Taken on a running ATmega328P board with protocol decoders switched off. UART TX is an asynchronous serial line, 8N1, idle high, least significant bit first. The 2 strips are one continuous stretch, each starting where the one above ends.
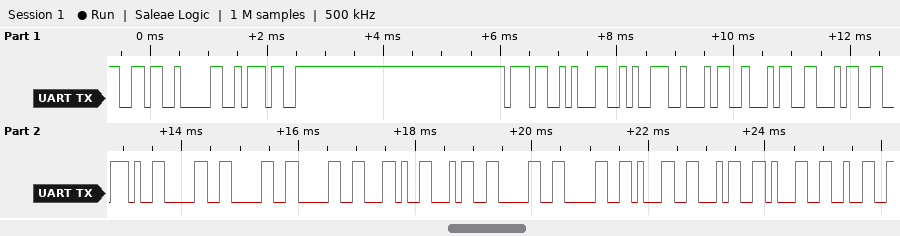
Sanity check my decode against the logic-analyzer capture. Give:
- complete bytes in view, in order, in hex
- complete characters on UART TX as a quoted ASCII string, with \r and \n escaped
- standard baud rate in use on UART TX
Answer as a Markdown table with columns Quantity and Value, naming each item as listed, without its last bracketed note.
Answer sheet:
| Quantity | Value |
|---|---|
| complete bytes in view, in order, in hex | 36 30 37 37 31 39 34 34 34 2E 30 30 30 2C 34 30 30 31 34 31 32 |
| complete characters on UART TX as a quoted ASCII string, with \r and \n escaped | "607719444.000,4001412" |
| standard baud rate in use on UART TX | 9600 baud |
